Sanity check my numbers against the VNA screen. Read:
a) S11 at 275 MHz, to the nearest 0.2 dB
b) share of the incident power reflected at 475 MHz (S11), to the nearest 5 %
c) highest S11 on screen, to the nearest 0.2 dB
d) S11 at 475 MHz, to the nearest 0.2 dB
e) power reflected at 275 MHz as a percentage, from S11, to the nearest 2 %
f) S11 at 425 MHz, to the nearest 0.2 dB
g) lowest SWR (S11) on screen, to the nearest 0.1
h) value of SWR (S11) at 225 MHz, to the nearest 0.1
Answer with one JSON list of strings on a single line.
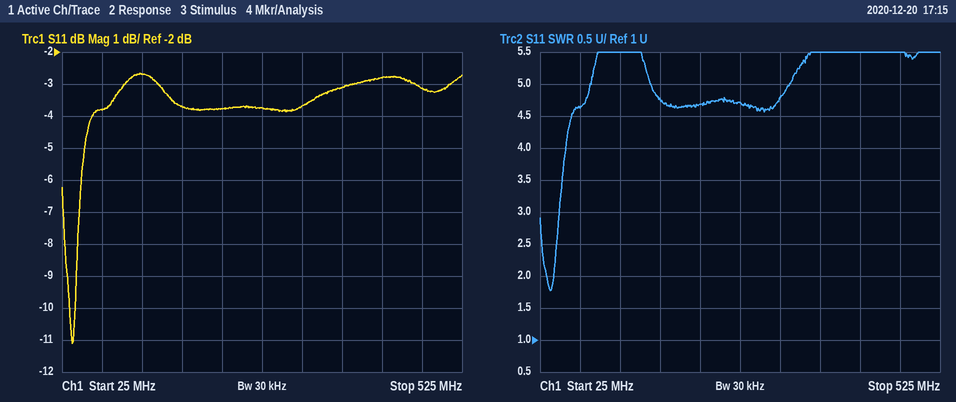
["-3.8 dB", "50 %", "-2.6 dB", "-3.2 dB", "42 %", "-2.8 dB", "1.8", "4.7"]
